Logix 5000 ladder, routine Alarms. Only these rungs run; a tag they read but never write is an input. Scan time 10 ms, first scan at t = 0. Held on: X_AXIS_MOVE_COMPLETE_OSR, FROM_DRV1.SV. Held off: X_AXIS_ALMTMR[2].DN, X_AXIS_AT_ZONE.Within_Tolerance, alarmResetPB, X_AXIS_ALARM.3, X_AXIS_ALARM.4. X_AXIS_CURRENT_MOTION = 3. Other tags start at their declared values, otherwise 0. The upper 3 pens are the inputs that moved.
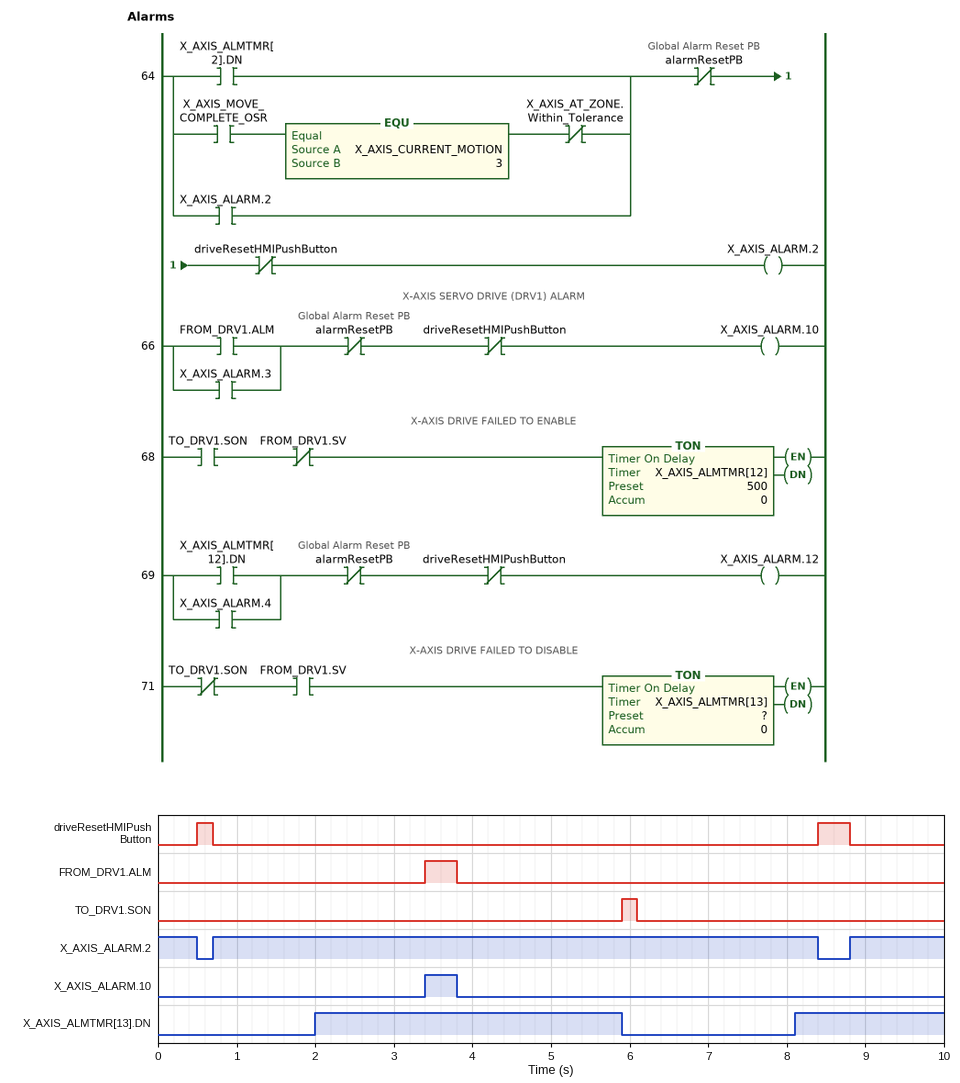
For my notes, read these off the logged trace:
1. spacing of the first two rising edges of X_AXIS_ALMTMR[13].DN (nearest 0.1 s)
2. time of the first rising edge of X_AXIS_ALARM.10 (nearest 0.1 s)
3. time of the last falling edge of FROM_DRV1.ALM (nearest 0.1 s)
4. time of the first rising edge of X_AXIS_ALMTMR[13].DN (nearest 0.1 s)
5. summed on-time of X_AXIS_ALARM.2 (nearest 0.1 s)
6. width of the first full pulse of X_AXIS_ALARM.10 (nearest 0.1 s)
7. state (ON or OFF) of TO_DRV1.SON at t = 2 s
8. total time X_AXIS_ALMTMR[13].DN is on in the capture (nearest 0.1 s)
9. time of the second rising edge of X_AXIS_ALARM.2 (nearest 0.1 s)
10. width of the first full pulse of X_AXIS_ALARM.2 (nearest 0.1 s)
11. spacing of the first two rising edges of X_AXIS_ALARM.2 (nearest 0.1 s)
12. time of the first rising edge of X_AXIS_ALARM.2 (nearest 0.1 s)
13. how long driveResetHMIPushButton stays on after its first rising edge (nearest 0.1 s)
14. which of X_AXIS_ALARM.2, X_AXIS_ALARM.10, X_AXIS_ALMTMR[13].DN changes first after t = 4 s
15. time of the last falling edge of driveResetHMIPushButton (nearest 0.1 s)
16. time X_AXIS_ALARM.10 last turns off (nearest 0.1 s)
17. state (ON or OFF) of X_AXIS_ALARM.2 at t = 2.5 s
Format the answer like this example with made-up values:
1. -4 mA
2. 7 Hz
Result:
1. 6.1 s
2. 3.4 s
3. 3.8 s
4. 2.0 s
5. 9.4 s
6. 0.4 s
7. OFF
8. 5.8 s
9. 8.8 s
10. 7.7 s
11. 8.1 s
12. 0.7 s
13. 0.2 s
14. X_AXIS_ALMTMR[13].DN
15. 8.8 s
16. 3.8 s
17. ON
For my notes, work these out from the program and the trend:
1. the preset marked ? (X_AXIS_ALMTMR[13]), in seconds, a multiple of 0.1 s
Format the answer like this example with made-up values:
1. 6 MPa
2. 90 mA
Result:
1. 2.0 s
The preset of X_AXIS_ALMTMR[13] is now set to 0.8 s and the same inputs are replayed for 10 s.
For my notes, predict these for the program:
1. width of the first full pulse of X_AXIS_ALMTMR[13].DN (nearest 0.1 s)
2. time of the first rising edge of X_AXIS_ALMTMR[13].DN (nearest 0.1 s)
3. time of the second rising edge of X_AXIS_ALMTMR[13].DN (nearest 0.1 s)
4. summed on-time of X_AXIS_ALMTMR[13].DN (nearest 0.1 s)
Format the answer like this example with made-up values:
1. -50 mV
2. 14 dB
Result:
1. 5.1 s
2. 0.8 s
3. 6.9 s
4. 8.2 s
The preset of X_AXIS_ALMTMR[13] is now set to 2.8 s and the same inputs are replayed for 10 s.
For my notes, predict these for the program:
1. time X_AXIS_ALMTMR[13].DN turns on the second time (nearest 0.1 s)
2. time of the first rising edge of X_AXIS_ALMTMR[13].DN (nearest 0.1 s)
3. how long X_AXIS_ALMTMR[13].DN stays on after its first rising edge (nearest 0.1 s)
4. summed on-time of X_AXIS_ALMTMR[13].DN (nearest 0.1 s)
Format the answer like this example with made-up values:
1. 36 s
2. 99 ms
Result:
1. 8.9 s
2. 2.8 s
3. 3.1 s
4. 4.2 s
